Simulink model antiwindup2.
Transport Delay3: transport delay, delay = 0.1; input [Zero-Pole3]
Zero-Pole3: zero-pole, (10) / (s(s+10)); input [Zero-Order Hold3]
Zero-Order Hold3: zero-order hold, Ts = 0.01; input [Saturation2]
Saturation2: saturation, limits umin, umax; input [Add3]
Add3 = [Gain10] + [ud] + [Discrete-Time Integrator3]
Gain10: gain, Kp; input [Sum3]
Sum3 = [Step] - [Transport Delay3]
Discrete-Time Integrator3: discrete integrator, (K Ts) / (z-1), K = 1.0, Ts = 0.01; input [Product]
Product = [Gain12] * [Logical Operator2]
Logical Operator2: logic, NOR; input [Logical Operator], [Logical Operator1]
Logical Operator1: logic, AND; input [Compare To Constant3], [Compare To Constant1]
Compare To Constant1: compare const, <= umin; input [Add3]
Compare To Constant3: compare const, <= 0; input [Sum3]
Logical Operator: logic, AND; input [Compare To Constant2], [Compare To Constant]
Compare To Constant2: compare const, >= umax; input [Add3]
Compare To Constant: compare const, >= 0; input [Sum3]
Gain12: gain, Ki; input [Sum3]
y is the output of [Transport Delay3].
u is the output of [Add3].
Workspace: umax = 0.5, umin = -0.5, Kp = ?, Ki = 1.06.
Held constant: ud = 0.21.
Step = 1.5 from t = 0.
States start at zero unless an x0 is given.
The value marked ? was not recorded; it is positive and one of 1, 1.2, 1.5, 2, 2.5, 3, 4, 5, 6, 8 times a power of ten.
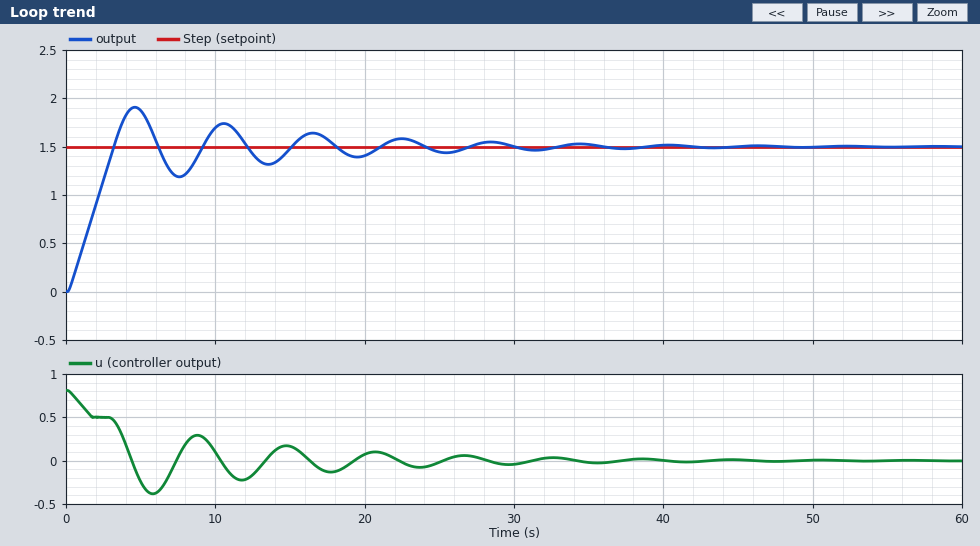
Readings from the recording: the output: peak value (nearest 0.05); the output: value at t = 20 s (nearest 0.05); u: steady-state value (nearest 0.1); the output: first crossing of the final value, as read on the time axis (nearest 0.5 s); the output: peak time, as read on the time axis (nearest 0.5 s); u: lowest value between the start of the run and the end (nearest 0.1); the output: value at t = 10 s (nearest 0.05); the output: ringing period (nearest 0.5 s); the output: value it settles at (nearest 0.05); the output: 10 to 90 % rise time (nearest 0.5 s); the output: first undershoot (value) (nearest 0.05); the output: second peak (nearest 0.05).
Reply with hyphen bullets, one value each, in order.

- 1.90
- 1.40
- 0.0
- 3.0 s
- 4.5 s
- -0.4
- 1.70
- 6.0 s
- 1.50
- 2.5 s
- 1.20
- 1.75
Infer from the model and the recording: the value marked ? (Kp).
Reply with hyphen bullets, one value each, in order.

- 0.4
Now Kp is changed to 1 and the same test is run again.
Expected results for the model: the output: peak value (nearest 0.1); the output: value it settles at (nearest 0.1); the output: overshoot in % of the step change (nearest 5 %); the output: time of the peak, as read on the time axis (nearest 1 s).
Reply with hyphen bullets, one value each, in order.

- 1.7
- 1.5
- 15 %
- 4 s
